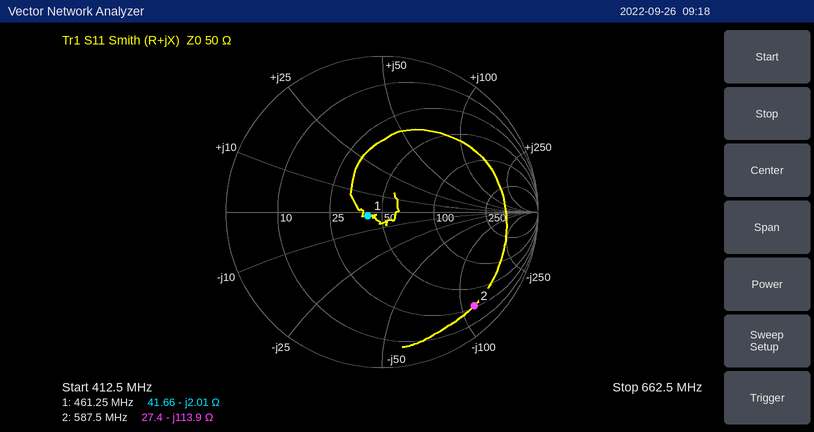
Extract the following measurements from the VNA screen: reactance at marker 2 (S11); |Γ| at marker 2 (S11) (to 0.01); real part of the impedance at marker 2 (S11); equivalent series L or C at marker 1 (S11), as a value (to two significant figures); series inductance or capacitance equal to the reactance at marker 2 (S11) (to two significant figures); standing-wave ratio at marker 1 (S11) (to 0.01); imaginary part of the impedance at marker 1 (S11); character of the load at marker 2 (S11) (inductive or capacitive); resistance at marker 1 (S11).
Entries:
-113.9 Ω
0.84
27.4 Ω
170 pF
2.4 pF
1.21
-2.01 Ω
capacitive
41.66 Ω
